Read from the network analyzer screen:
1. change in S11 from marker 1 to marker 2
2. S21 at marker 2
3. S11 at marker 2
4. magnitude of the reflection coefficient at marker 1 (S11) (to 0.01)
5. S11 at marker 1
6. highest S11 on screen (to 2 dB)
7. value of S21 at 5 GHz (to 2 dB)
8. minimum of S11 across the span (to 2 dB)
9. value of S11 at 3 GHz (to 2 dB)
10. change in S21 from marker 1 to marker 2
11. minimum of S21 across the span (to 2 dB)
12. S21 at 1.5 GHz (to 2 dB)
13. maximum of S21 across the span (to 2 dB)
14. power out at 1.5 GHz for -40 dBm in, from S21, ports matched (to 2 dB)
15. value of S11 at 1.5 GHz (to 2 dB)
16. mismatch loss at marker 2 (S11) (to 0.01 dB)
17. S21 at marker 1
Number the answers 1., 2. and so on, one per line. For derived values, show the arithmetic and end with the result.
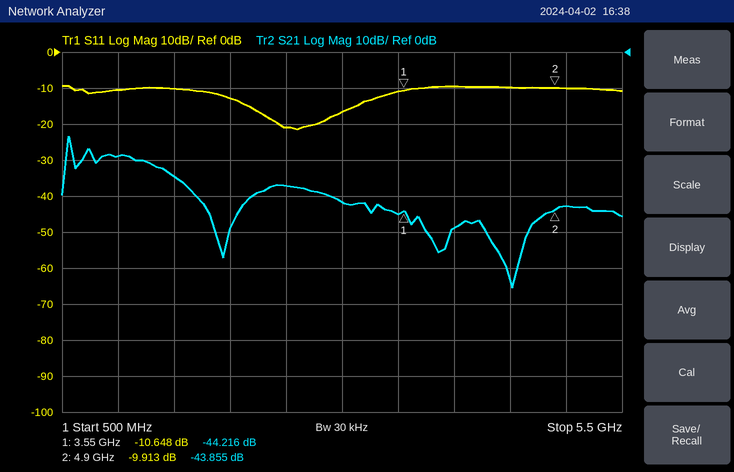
1. -9.913 − (-10.648) = 0.735 dB
2. -43.855 dB
3. -9.913 dB
4. 10^(-10.648/20) ≈ 0.29
5. -10.648 dB
6. -10 dB
7. -42 dB
8. -22 dB
9. -16 dB
10. -43.855 − (-44.216) = 0.361 dB
11. -66 dB
12. -34 dB
13. -24 dB
14. -40 dBm + (-34 dB) = -74 dBm
15. -10 dB
16. −10 log10(1 − 10^(-9.913/10)) ≈ 0.47 dB
17. -44.216 dB
